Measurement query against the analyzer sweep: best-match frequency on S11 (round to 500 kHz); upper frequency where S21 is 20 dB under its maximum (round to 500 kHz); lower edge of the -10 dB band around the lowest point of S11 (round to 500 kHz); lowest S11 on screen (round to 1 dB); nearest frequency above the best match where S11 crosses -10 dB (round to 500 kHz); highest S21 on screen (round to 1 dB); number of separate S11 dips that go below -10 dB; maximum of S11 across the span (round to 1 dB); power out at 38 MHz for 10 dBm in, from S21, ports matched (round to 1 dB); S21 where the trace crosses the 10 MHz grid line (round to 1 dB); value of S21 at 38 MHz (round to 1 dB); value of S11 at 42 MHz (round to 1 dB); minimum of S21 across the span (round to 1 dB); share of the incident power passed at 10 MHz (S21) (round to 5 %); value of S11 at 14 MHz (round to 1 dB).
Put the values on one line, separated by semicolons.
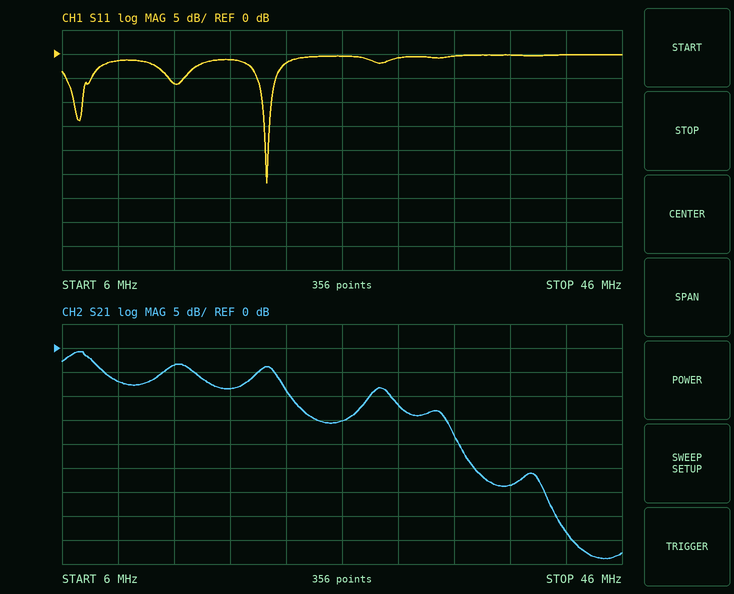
20.5 MHz; 34.5 MHz; 20.5 MHz; -27 dB; 21.0 MHz; -1 dB; 2; 0 dB; -19 dBm; -7 dB; -29 dB; 0 dB; -44 dB; 20 %; -6 dB
